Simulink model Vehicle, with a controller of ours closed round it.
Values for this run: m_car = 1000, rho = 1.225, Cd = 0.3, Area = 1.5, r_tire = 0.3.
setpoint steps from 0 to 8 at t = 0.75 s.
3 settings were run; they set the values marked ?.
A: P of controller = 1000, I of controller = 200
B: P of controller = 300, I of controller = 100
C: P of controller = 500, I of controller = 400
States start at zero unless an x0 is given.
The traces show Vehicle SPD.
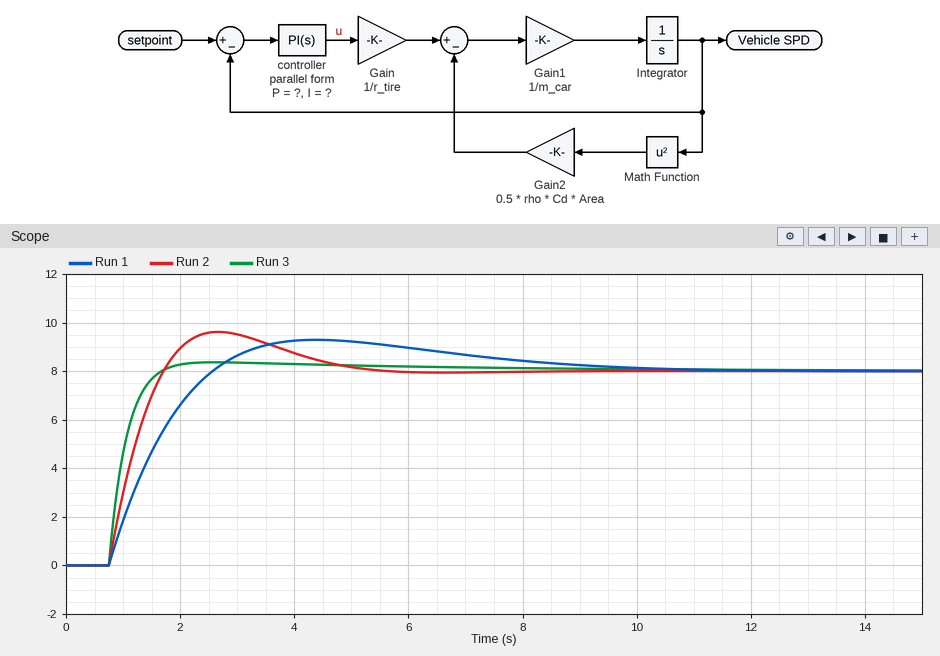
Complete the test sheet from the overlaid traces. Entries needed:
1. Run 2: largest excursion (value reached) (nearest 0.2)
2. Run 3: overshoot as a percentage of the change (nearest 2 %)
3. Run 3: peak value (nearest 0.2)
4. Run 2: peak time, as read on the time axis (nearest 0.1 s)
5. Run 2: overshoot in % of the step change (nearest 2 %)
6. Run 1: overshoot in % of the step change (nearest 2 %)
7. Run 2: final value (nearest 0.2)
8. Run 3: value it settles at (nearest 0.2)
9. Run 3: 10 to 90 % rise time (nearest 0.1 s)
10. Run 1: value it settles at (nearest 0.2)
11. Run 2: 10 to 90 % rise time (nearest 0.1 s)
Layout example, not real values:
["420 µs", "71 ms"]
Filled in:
["9.6", "4 %", "8.4", "2.7 s", "20 %", "16 %", "8.0", "8.0", "0.6 s", "8.0", "0.7 s"]
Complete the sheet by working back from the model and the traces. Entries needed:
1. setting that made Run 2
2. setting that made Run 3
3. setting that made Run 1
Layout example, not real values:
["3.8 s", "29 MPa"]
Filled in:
["C", "A", "B"]
